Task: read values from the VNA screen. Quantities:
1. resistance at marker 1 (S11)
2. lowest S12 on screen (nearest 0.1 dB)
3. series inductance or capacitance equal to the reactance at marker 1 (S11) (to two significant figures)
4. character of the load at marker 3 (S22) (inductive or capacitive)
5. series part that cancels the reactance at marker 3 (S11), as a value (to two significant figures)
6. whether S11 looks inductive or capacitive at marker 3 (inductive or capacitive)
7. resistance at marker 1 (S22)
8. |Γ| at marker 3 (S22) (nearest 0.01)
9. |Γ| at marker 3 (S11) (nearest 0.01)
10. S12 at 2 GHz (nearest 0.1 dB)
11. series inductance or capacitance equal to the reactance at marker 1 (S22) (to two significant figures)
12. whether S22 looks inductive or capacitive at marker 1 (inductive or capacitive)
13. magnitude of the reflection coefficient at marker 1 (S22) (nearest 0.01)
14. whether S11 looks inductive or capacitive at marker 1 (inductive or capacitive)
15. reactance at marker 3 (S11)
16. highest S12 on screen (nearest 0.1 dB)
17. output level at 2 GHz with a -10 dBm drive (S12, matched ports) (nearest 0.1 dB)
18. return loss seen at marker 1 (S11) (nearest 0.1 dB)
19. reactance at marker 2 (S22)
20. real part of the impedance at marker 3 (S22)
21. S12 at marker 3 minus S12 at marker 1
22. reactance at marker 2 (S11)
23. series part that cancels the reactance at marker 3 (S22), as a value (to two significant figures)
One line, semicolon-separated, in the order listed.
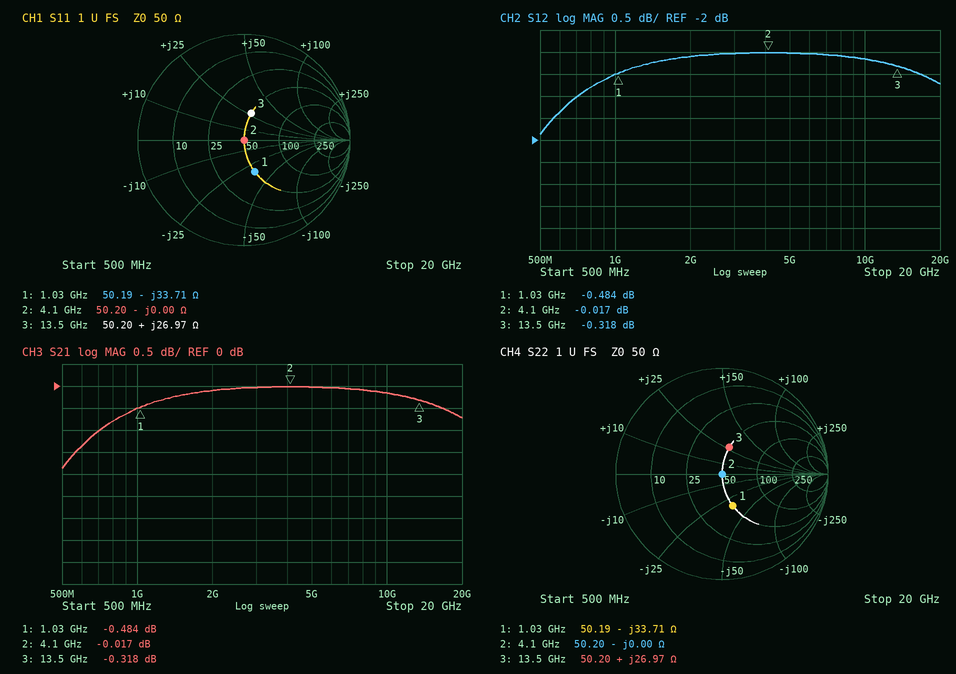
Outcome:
50.19 Ω; -1.9 dB; 4.6 pF; inductive; 440 fF; inductive; 50.19 Ω; 0.26; 0.26; -0.1 dB; 4.6 pF; capacitive; 0.32; capacitive; +26.97 Ω; 0.0 dB; -10.1 dBm; 9.9 dB; -0.00 Ω; 50.20 Ω; 0.166 dB; -0.00 Ω; 440 fF
